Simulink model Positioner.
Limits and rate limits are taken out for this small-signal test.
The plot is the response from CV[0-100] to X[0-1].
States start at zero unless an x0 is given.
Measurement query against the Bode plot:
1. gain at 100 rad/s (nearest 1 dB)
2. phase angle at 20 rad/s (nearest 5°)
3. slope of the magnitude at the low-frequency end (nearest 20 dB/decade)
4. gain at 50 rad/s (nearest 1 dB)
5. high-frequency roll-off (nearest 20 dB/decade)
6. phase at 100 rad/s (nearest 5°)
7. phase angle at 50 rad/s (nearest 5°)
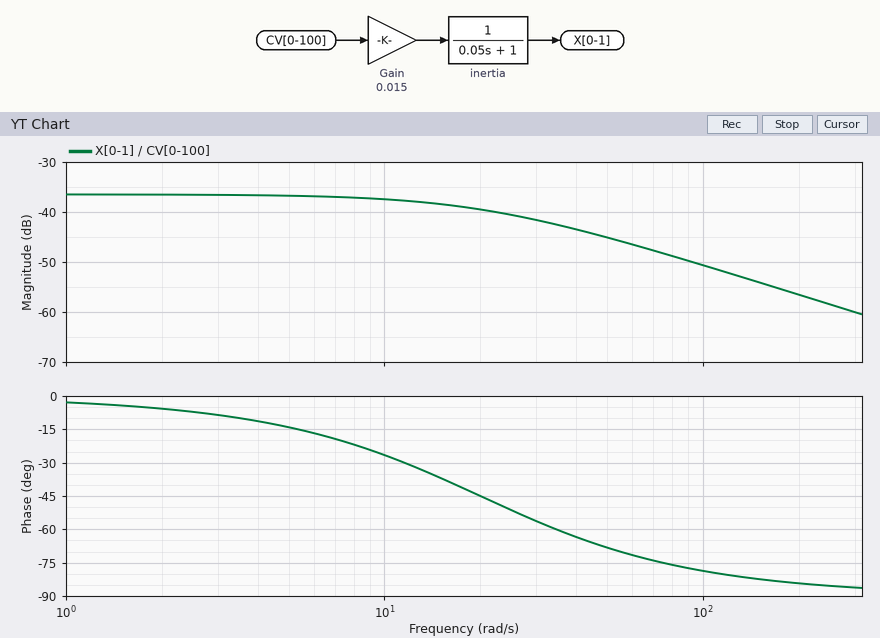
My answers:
-51 dB
-45°
0 dB/decade
-45 dB
-20 dB/decade
-80°
-70°
